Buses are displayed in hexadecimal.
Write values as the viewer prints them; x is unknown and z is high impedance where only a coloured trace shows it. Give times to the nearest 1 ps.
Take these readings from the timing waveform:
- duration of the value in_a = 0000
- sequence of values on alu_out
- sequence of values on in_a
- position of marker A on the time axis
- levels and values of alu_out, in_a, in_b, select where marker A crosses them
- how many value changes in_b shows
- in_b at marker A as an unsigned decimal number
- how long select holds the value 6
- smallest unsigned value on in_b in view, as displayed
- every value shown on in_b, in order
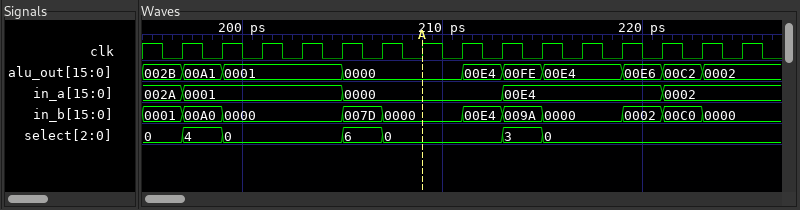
8 ps
002B, 00A1, 0001, 0000, 00E4, 00FE, 00E4, 00E6, 00C2, 0002
002A, 0001, 0000, 00E4, 0002
209 ps
alu_out=0000, in_a=0000, in_b=0000, select=0
10
0
2 ps
0000
0001, 00A0, 0000, 007D, 0000, 00E4, 009A, 0000, 0002, 00C0, 0000
